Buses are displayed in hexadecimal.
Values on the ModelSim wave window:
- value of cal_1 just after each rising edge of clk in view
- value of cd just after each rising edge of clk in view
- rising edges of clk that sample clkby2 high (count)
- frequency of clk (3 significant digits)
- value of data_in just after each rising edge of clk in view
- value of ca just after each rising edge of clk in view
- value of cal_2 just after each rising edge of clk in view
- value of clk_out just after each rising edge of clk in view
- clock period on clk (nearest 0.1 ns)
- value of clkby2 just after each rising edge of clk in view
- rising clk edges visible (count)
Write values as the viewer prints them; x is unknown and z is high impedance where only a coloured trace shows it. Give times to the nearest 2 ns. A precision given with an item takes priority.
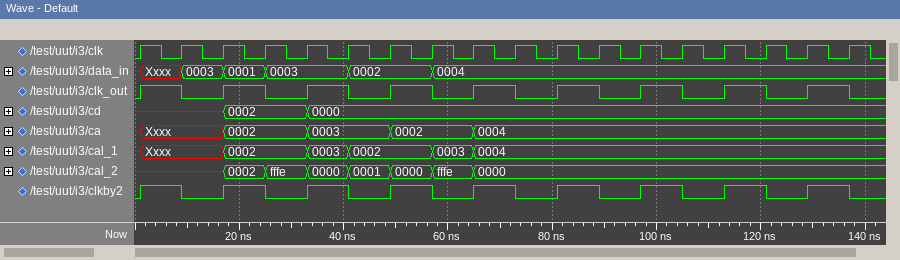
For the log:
Xxxx, Xxxx, 0002, 0002, 0003, 0002, 0002, 0003, 0004, 0004, 0004, 0004, 0004, 0004, 0004, 0004, 0004, 0004
x, x, 0002, 0002, 0000, 0000, 0000, 0000, 0000, 0000, 0000, 0000, 0000, 0000, 0000, 0000, 0000, 0000
9
125 MHz
Xxxx, 0003, 0001, 0003, 0003, 0002, 0002, 0004, 0004, 0004, 0004, 0004, 0004, 0004, 0004, 0004, 0004, 0004
Xxxx, Xxxx, 0002, 0002, 0003, 0003, 0002, 0002, 0004, 0004, 0004, 0004, 0004, 0004, 0004, 0004, 0004, 0004
x, x, 0002, fffe, 0000, 0001, 0000, fffe, 0000, 0000, 0000, 0000, 0000, 0000, 0000, 0000, 0000, 0000
1 0 1 0 1 0 1 0 1 0 1 0 1 0 1 0 1 0
8 ns
1 0 1 0 1 0 1 0 1 0 1 0 1 0 1 0 1 0
18
